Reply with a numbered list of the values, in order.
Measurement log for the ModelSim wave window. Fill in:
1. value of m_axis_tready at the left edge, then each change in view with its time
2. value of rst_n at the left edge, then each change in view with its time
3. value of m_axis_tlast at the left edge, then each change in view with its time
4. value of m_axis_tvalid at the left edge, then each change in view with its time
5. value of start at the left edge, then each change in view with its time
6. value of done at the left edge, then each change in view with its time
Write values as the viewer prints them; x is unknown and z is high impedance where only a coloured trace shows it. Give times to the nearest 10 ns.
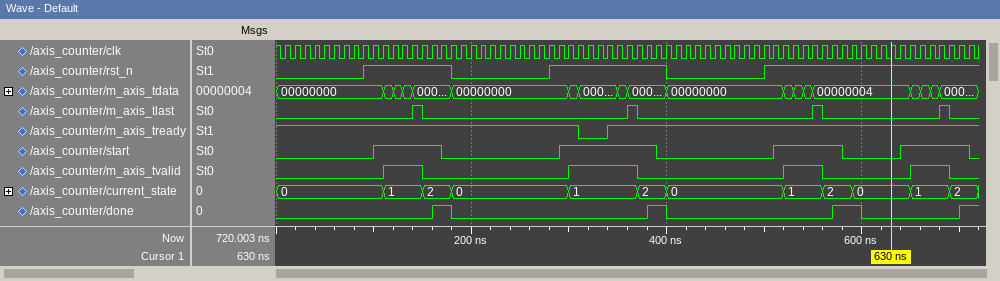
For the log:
1. 1, 0 at 310 ns, 1 at 340 ns
2. 0, 1 at 90 ns, 0 at 180 ns, 1 at 280 ns, 0 at 400 ns, 1 at 500 ns
3. 0, 1 at 140 ns, 0 at 150 ns, 1 at 360 ns, 0 at 370 ns, 1 at 550 ns, 0 at 560 ns, 1 at 680 ns, 0 at 690 ns
4. 0, 1 at 110 ns, 0 at 150 ns, 1 at 300 ns, 0 at 370 ns, 1 at 520 ns, 0 at 560 ns, 1 at 650 ns, 0 at 690 ns
5. 0, 1 at 100 ns, 0 at 170 ns, 1 at 290 ns, 0 at 390 ns, 1 at 510 ns, 0 at 580 ns, 1 at 640 ns, 0 at 710 ns
6. 0, 1 at 160 ns, 0 at 180 ns, 1 at 380 ns, 0 at 400 ns, 1 at 570 ns, 0 at 600 ns, 1 at 700 ns
